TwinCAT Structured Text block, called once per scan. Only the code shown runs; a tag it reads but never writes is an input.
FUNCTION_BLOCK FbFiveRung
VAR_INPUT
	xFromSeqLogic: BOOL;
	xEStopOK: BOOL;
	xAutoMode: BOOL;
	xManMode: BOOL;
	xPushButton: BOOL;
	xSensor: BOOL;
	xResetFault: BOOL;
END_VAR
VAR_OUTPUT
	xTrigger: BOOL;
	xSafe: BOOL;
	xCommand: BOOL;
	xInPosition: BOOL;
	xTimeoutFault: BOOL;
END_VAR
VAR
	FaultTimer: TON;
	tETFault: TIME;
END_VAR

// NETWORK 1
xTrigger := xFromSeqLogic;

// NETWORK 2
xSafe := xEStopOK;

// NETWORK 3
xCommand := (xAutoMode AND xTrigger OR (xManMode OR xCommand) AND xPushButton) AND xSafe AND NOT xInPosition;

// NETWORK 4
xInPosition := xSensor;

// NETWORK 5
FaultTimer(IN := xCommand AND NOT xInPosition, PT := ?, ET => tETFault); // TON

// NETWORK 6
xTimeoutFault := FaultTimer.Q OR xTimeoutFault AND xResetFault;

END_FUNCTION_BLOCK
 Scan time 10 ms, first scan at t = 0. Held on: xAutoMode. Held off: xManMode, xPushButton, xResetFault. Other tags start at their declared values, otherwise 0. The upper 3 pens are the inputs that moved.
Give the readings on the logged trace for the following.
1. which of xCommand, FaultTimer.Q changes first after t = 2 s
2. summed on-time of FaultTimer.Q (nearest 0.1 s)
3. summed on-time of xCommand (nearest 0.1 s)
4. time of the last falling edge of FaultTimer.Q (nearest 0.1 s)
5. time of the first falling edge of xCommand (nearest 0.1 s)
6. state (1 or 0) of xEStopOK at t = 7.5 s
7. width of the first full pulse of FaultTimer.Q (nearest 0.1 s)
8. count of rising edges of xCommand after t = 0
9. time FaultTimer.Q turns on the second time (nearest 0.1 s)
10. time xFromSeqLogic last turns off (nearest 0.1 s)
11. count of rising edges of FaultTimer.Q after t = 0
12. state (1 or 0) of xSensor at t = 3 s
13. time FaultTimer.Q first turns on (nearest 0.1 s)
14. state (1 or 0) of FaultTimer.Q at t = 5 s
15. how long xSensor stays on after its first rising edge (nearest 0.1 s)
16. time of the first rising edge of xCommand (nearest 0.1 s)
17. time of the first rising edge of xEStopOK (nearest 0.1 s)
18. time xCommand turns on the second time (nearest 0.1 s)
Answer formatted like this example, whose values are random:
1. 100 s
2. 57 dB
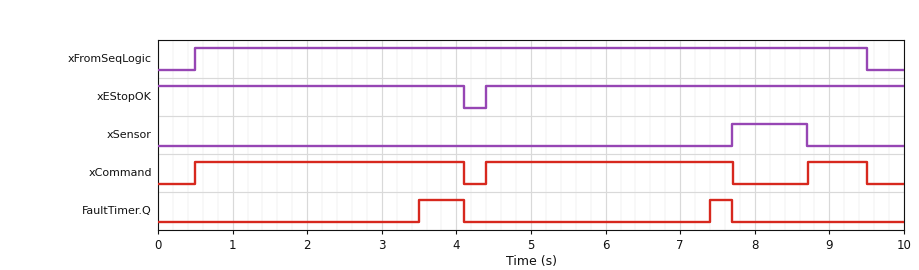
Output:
1. FaultTimer.Q
2. 0.9 s
3. 7.7 s
4. 7.7 s
5. 4.1 s
6. 1
7. 0.6 s
8. 3
9. 7.4 s
10. 9.5 s
11. 2
12. 0
13. 3.5 s
14. 0
15. 1.0 s
16. 0.5 s
17. 4.4 s
18. 4.4 s
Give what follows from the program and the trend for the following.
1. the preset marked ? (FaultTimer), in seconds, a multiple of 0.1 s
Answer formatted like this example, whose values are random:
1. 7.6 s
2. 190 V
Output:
1. 3.0 s
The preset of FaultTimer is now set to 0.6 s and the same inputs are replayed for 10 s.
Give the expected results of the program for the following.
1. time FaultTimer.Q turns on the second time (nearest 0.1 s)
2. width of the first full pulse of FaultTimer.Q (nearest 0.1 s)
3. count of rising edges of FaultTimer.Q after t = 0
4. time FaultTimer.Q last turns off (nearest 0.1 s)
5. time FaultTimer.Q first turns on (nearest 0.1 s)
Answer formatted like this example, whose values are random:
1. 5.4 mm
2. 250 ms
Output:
1. 5.0 s
2. 3.0 s
3. 3
4. 9.5 s
5. 1.1 s
